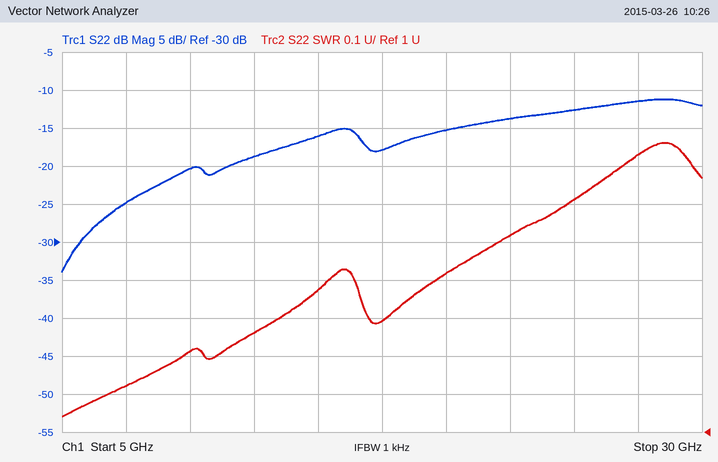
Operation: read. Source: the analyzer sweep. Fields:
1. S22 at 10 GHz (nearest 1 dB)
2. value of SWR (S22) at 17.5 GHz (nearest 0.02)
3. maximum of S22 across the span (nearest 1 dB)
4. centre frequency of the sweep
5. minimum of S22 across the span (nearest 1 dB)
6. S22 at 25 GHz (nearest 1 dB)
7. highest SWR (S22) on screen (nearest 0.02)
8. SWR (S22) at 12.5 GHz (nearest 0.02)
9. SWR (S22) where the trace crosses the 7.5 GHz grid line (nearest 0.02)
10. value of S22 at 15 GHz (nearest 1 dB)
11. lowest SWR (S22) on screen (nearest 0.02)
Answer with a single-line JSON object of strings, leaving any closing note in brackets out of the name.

{"S22 at 10 GHz": "-20 dB", "value of SWR (S22) at 17.5 GHz": "1.30", "maximum of S22 across the span": "-11 dB", "centre frequency of the sweep": "17.5 GHz", "minimum of S22 across the span": "-34 dB", "S22 at 25 GHz": "-13 dB", "highest SWR (S22) on screen": "1.76", "SWR (S22) at 12.5 GHz": "1.26", "SWR (S22) where the trace crosses the 7.5 GHz grid line": "1.12", "value of S22 at 15 GHz": "-16 dB", "lowest SWR (S22) on screen": "1.04"}
